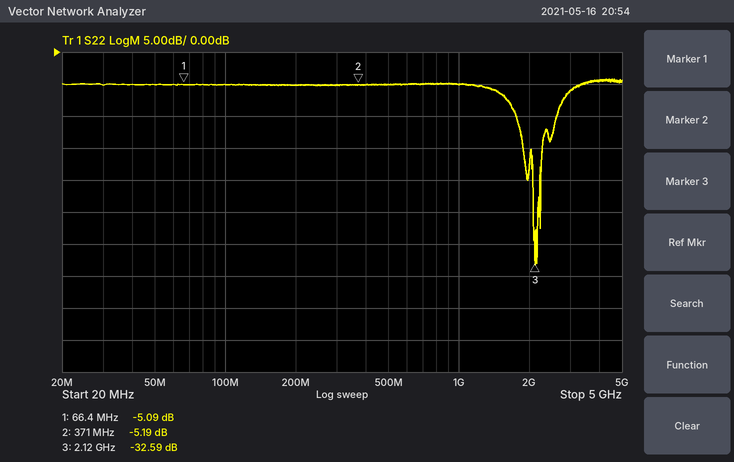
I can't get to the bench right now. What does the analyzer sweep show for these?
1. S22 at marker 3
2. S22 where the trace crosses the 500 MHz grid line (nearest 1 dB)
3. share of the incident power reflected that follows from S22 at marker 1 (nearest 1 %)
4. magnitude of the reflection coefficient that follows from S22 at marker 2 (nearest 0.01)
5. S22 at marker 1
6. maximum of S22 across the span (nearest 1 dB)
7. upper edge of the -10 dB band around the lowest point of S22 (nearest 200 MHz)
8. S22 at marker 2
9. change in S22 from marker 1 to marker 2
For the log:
-32.59 dB
-5 dB
31 %
0.55
-5.09 dB
-4 dB
2.6 GHz
-5.19 dB
-0.10 dB
